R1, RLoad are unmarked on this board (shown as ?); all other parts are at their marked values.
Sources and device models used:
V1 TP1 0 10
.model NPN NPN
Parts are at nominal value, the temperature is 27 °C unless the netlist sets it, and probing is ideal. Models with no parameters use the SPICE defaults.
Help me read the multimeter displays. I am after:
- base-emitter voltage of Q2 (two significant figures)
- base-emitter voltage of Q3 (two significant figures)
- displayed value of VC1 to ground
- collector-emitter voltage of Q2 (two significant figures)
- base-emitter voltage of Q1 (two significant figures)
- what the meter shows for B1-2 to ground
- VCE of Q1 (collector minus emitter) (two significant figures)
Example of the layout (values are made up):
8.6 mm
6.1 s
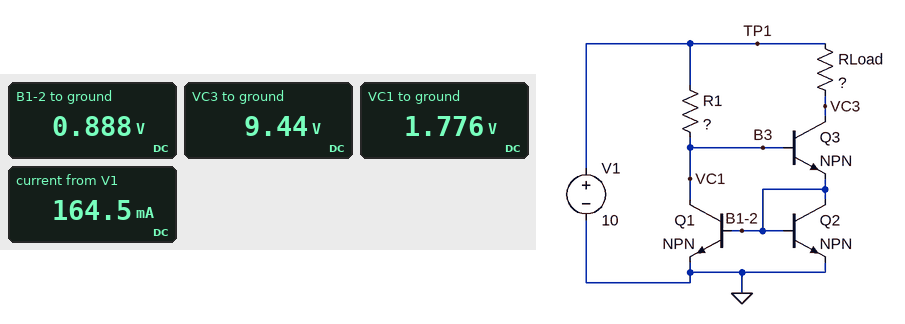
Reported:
890 mV
890 mV
1.776 V
890 mV
890 mV
0.888 V
1.8 V
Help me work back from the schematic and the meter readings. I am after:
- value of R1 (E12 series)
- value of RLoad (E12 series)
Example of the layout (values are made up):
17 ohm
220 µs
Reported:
100 Ω
6.8 Ω
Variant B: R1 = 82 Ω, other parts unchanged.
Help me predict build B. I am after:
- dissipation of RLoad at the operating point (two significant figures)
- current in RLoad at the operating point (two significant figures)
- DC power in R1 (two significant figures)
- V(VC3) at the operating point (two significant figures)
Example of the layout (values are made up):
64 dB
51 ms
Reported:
68 mW
100 mA
820 mW
9.3 V
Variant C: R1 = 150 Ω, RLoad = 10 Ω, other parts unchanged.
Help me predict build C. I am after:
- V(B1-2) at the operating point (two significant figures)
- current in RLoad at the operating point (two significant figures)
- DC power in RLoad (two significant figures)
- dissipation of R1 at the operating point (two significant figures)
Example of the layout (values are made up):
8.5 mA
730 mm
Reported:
880 mV
55 mA
30 mW
450 mW
